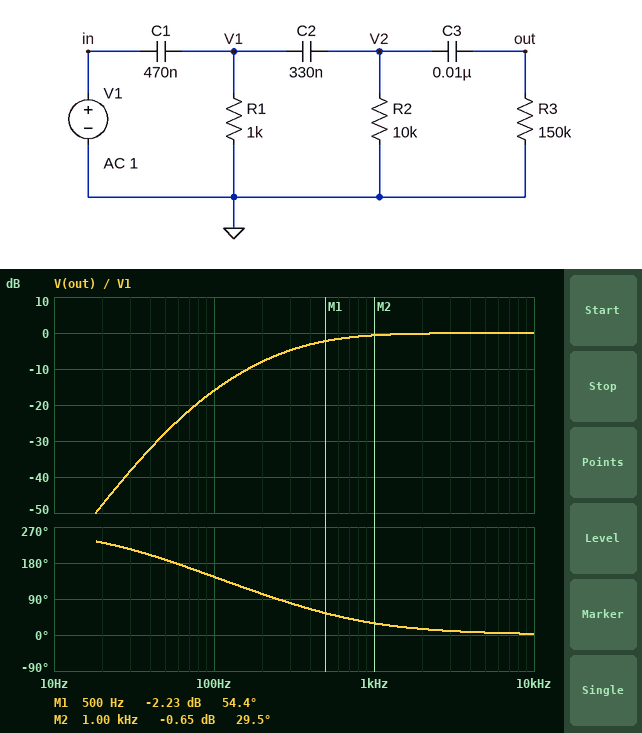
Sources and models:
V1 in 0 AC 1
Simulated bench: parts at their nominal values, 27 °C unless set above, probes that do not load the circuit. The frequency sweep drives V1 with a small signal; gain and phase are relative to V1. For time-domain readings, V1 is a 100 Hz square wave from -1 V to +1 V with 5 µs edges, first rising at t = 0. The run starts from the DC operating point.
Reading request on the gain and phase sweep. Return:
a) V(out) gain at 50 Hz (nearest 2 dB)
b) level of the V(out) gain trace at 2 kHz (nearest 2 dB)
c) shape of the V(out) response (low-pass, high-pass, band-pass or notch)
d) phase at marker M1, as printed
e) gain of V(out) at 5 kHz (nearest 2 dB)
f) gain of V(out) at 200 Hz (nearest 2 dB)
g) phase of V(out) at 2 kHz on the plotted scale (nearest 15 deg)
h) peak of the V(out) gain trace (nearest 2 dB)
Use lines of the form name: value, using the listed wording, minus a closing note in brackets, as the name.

V(out) gain at 50 Hz: -28 dB
level of the V(out) gain trace at 2 kHz: 0 dB
shape of the V(out) response: high-pass
phase at marker M1, as printed: 54.4 deg
gain of V(out) at 5 kHz: 0 dB
gain of V(out) at 200 Hz: -8 dB
phase of V(out) at 2 kHz on the plotted scale: 15 deg
peak of the V(out) gain trace: 0 dB
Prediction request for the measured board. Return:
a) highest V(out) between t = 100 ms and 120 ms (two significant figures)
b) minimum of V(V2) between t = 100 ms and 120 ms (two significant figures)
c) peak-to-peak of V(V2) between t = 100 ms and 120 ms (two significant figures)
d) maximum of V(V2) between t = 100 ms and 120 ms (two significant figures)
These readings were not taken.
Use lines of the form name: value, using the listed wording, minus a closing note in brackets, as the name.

highest V(out) between t = 100 ms and 120 ms: 2.0 V
minimum of V(V2) between t = 100 ms and 120 ms: -2.0 V
peak-to-peak of V(V2) between t = 100 ms and 120 ms: 4.1 V
maximum of V(V2) between t = 100 ms and 120 ms: 2.0 V
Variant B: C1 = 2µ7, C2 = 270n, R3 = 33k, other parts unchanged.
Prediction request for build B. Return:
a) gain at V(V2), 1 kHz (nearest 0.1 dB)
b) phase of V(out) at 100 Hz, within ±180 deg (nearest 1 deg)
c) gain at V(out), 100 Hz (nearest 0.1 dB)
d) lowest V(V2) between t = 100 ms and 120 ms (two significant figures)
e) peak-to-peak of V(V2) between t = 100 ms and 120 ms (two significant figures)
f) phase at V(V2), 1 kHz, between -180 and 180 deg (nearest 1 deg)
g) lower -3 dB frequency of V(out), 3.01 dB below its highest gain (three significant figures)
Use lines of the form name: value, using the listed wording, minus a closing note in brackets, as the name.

gain at V(V2), 1 kHz: -0.1 dB
phase of V(out) at 100 Hz, within ±180 deg: 140 deg
gain at V(out), 100 Hz: -17.0 dB
lowest V(V2) between t = 100 ms and 120 ms: -2.1 V
peak-to-peak of V(V2) between t = 100 ms and 120 ms: 4.3 V
phase at V(V2), 1 kHz, between -180 and 180 deg: 8 deg
lower -3 dB frequency of V(out), 3.01 dB below its highest gain: 520 Hz
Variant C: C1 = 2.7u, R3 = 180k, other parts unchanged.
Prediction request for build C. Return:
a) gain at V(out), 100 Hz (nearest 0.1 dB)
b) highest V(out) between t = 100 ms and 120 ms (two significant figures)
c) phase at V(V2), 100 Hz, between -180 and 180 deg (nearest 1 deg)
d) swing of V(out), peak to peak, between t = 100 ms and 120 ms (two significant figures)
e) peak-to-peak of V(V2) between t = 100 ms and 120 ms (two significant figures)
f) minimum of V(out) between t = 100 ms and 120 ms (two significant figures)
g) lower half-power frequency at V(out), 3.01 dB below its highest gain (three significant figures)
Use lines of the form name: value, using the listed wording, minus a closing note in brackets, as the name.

gain at V(out), 100 Hz: -5.2 dB
highest V(out) between t = 100 ms and 120 ms: 2.2 V
phase at V(V2), 100 Hz, between -180 and 180 deg: 58 deg
swing of V(out), peak to peak, between t = 100 ms and 120 ms: 4.5 V
peak-to-peak of V(V2) between t = 100 ms and 120 ms: 4.2 V
minimum of V(out) between t = 100 ms and 120 ms: -2.2 V
lower half-power frequency at V(out), 3.01 dB below its highest gain: 139 Hz
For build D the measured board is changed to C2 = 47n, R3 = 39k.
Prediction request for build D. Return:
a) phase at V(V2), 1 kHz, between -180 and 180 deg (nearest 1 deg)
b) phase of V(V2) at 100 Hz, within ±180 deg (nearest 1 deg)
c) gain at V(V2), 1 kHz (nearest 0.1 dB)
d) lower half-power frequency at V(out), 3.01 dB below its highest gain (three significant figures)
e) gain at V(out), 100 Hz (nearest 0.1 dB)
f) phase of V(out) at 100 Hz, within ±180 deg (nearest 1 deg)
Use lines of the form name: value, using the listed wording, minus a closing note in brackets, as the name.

phase at V(V2), 1 kHz, between -180 and 180 deg: 42 deg
phase of V(V2) at 100 Hz, within ±180 deg: 143 deg
gain at V(V2), 1 kHz: -1.6 dB
lower half-power frequency at V(out), 3.01 dB below its highest gain: 846 Hz
gain at V(out), 100 Hz: -34.8 dB
phase of V(out) at 100 Hz, within ±180 deg: -141 deg
